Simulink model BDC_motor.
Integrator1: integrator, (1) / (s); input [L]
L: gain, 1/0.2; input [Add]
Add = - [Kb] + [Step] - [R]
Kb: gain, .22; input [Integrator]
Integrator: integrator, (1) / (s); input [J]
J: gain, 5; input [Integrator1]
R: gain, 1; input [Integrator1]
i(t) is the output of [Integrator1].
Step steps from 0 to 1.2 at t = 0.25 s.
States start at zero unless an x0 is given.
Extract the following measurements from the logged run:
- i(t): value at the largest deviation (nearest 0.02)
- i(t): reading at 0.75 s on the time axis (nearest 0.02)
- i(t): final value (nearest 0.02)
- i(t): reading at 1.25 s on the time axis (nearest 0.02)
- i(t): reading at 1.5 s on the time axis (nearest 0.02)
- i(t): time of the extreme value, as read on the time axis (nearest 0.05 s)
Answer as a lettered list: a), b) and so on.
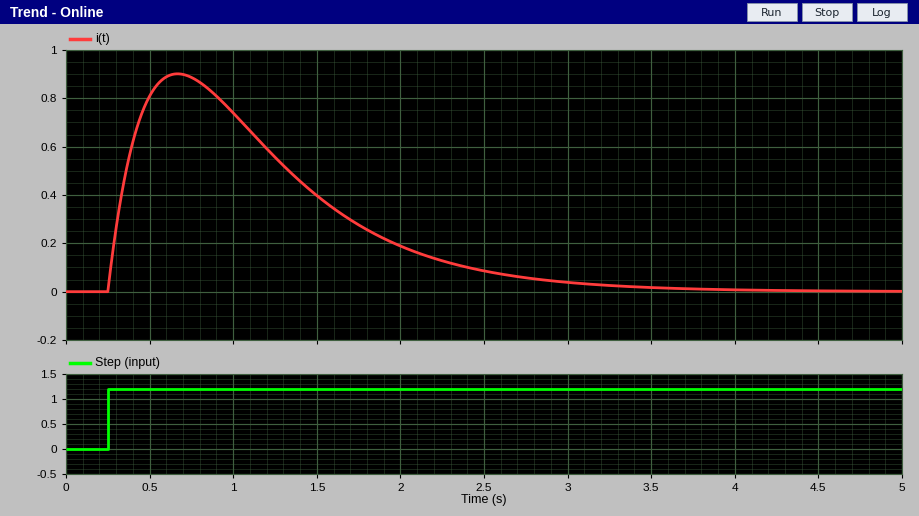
a) 0.90
b) 0.88
c) 0.00
d) 0.56
e) 0.40
f) 0.65 s
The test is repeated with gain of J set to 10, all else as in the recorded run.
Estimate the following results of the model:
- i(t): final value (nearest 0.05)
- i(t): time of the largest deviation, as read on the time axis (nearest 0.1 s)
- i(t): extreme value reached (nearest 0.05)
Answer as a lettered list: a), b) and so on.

a) 0.00
b) 0.6 s
c) 0.80
